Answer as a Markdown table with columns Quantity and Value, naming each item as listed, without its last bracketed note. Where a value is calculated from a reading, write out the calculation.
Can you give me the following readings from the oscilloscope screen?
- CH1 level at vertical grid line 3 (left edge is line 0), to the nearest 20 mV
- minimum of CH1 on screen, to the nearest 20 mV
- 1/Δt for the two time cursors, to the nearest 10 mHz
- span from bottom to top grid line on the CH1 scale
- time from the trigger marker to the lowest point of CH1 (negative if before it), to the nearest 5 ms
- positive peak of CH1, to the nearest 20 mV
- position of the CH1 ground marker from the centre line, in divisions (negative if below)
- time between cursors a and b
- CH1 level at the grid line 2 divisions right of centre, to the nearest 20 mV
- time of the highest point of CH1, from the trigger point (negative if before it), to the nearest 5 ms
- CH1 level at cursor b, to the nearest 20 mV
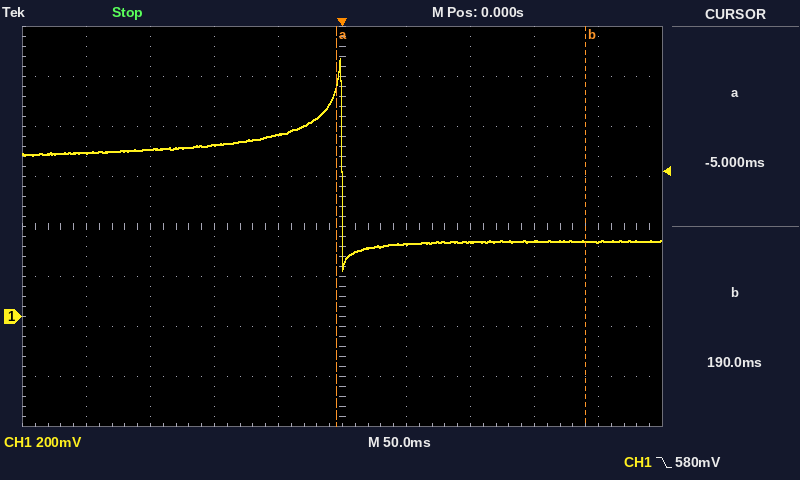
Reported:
| Quantity | Value |
|---|---|
| CH1 level at vertical grid line 3 (left edge is line 0), to the nearest 20 mV | 680 mV |
| minimum of CH1 on screen, to the nearest 20 mV | 180 mV |
| 1/Δt for the two time cursors, to the nearest 10 mHz | 1 / 195 ms ≈ 5.13 Hz |
| span from bottom to top grid line on the CH1 scale | 1.6 V |
| time from the trigger marker to the lowest point of CH1 (negative if before it), to the nearest 5 ms | 0 ms |
| positive peak of CH1, to the nearest 20 mV | 1.04 V |
| position of the CH1 ground marker from the centre line, in divisions | -1.8 div |
| time between cursors a and b | 190 ms − (-5 ms) = 195 ms |
| CH1 level at the grid line 2 divisions right of centre, to the nearest 20 mV | 300 mV |
| time of the highest point of CH1, from the trigger point (negative if before it), to the nearest 5 ms | 0 ms |
| CH1 level at cursor b, to the nearest 20 mV | 300 mV |
